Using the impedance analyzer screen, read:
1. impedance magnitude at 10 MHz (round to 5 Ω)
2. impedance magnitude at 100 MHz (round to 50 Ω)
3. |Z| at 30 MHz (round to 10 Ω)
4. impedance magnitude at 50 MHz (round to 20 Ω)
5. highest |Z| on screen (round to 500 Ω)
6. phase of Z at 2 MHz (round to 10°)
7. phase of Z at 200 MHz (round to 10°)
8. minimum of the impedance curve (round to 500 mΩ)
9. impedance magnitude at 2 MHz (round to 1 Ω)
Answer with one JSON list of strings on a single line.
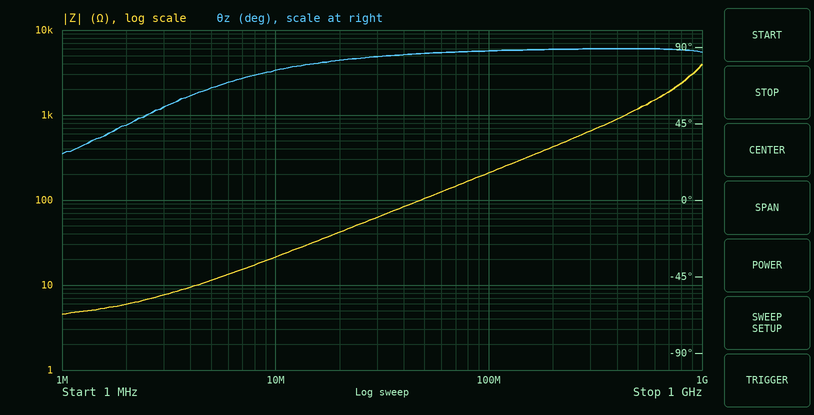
["20 Ω", "200 Ω", "60 Ω", "100 Ω", "4.0 kΩ", "40°", "90°", "4.5 Ω", "6 Ω"]
